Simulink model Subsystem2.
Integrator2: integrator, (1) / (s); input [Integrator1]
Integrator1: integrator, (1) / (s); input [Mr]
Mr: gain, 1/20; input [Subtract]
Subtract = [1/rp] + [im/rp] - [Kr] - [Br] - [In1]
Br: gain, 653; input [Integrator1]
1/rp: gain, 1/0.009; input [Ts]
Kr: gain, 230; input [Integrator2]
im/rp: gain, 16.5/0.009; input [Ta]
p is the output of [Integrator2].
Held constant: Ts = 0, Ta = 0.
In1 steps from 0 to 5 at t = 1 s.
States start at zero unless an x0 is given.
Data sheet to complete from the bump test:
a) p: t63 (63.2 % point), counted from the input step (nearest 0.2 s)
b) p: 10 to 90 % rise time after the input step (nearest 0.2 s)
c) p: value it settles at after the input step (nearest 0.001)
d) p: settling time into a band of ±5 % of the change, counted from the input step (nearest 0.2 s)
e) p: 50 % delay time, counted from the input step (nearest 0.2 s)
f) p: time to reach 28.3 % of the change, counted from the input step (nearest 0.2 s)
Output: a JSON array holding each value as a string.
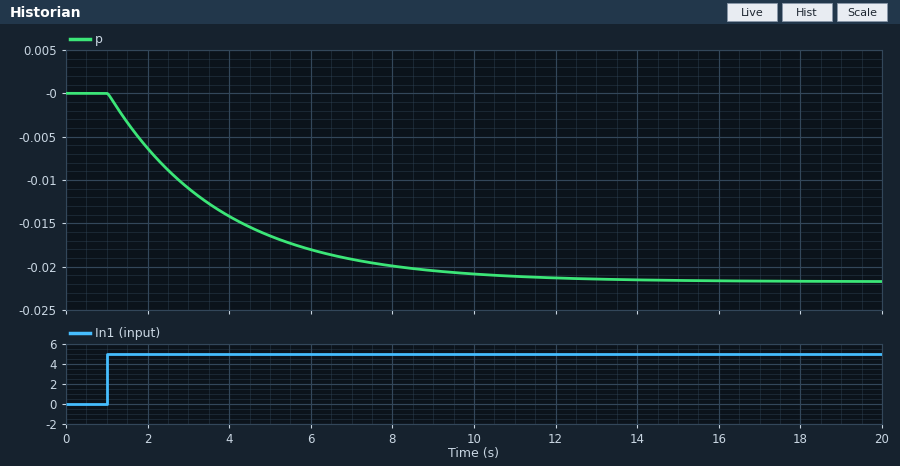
["2.8 s", "6.2 s", "-0.022", "8.4 s", "2.0 s", "1.0 s"]
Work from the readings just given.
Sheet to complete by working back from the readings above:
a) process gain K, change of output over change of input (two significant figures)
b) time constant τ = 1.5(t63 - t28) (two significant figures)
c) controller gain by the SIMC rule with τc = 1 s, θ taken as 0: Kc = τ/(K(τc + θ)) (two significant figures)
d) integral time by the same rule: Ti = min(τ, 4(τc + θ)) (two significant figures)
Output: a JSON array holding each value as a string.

["-0.0044", "2.7 s", "-610", "2.7 s"]
